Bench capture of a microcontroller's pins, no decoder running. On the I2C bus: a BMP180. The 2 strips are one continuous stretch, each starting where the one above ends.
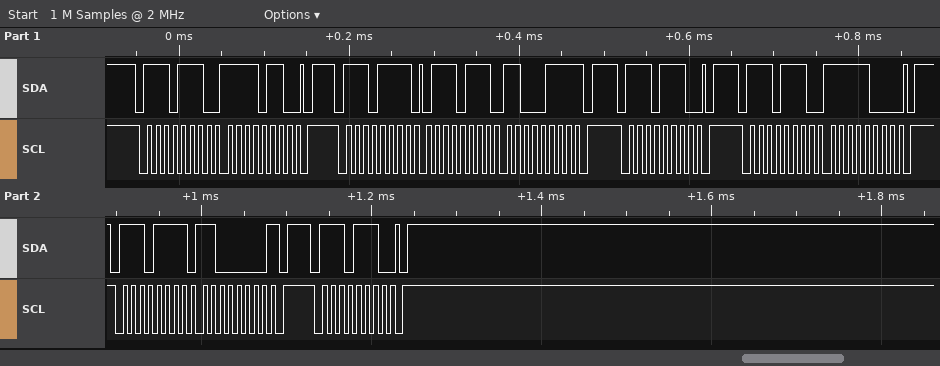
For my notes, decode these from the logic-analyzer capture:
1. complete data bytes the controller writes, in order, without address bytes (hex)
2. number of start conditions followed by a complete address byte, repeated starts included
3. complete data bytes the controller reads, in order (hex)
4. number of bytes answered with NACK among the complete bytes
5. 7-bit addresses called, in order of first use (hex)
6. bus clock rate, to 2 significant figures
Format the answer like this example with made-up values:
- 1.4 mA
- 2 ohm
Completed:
- F6 F8
- 6
- 77 C7 C0
- 2
- 0x77
- 100 kHz
